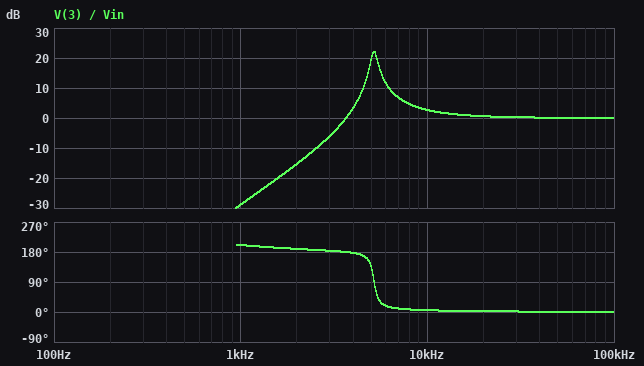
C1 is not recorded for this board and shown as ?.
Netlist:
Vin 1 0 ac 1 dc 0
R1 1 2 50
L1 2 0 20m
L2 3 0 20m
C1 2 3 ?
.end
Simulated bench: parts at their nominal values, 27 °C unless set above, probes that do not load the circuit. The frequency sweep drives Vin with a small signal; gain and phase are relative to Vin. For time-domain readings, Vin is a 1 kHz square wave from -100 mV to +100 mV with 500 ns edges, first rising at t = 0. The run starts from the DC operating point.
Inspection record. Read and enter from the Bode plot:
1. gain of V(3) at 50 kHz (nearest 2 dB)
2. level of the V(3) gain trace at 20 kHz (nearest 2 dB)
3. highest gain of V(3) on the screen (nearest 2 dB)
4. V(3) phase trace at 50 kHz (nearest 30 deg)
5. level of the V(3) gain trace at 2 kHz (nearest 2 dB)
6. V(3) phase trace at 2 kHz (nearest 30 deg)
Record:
0 dB
0 dB
22 dB
0 deg
-16 dB
180 deg
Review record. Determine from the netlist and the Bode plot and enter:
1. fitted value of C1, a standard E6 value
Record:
47 nF
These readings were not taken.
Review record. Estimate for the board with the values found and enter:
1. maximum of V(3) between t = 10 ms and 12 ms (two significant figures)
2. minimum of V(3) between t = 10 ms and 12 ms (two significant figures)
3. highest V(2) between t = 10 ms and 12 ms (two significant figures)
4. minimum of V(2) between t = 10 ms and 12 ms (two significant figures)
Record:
300 mV
-300 mV
140 mV
-140 mV
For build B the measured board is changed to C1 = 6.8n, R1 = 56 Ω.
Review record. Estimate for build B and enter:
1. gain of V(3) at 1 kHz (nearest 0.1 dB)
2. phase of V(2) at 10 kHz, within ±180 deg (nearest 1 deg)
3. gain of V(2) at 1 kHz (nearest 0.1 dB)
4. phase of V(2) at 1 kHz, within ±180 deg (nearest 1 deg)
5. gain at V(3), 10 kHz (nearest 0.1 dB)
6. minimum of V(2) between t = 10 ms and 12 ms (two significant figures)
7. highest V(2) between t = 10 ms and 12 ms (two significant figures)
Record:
-46.1 dB
0 deg
-0.8 dB
24 deg
1.3 dB
-160 mV
160 mV
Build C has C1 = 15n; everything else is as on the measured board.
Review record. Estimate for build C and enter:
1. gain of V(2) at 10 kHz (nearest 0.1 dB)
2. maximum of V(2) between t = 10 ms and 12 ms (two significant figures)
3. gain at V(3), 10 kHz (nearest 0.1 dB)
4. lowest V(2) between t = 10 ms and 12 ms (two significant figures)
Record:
-0.4 dB
150 mV
15.8 dB
-150 mV
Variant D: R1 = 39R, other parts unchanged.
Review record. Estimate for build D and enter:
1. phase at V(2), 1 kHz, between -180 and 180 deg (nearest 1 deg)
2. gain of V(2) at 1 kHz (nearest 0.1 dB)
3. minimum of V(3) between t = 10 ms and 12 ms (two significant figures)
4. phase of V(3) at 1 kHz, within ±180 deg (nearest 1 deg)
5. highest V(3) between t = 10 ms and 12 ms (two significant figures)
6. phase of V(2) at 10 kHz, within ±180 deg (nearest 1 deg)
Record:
17 deg
-0.4 dB
-320 mV
-163 deg
320 mV
4 deg
